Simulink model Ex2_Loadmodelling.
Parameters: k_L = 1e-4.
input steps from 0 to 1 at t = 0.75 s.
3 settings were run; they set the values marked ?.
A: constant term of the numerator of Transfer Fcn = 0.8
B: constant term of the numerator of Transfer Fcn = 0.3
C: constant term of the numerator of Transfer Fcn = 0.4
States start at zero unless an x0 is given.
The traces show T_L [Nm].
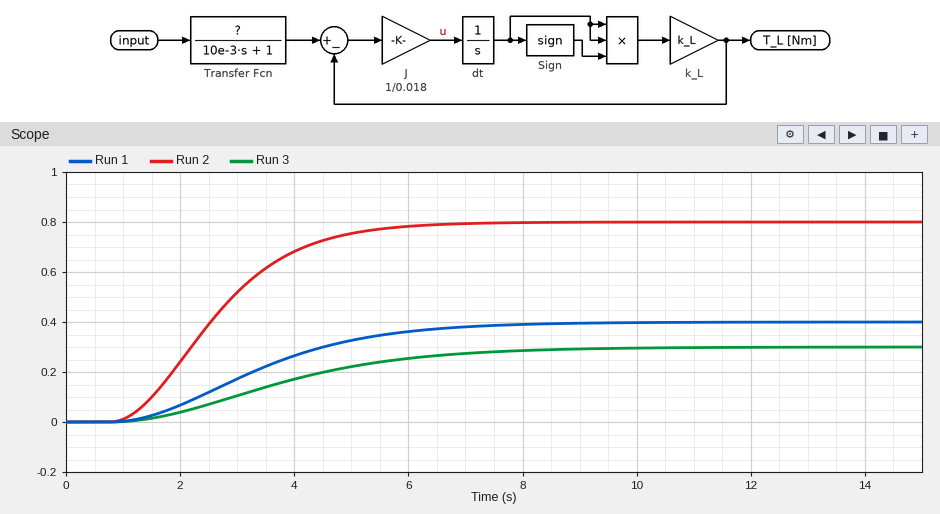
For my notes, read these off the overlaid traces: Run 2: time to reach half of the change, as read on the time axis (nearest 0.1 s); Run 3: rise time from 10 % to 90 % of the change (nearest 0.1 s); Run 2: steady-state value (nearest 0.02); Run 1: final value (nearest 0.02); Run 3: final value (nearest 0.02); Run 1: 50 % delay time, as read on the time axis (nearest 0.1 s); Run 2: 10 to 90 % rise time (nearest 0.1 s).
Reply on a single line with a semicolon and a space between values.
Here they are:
2.5 s; 4.9 s; 0.80; 0.40; 0.30; 3.3 s; 3.0 s
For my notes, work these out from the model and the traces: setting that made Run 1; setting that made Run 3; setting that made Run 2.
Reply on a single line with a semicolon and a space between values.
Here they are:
C; B; A
